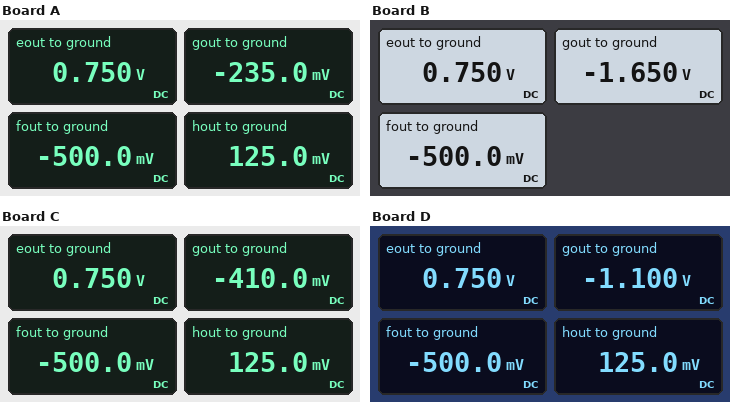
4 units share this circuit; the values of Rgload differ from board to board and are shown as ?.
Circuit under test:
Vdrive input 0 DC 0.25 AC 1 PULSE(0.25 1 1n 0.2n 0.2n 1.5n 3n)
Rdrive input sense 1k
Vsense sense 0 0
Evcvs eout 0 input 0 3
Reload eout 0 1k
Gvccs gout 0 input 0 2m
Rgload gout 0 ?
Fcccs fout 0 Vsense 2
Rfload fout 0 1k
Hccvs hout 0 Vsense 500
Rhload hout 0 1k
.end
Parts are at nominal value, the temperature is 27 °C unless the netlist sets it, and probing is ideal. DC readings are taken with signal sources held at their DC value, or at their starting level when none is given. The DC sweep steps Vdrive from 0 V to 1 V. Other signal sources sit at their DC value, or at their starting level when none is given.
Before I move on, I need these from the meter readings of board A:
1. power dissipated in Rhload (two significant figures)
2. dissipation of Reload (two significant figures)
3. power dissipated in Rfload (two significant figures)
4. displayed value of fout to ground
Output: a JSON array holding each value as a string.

["16 µW", "560 µW", "250 µW", "-500.0 mV"]
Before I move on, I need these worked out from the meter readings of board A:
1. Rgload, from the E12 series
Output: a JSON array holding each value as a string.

["470 Ω"]
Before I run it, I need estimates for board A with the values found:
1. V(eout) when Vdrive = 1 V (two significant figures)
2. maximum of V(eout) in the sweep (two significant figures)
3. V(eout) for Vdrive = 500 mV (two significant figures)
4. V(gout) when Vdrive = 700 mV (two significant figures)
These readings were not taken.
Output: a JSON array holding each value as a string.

["3.0 V", "3.0 V", "1.5 V", "-660 mV"]
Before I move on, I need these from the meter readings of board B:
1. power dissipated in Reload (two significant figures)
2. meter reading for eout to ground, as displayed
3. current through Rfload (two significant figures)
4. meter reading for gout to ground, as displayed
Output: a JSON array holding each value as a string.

["560 µW", "0.750 V", "500 µA", "-1.650 V"]
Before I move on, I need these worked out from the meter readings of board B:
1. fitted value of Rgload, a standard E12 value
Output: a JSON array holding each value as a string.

["3.3 kΩ"]
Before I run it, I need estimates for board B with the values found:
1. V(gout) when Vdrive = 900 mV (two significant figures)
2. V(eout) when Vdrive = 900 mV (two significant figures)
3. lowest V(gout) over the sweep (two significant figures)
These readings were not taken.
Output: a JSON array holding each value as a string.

["-5.9 V", "2.7 V", "-6.6 V"]
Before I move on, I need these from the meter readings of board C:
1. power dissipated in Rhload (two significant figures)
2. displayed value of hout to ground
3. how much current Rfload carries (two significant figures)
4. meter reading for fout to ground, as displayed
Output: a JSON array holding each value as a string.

["16 µW", "125.0 mV", "500 µA", "-500.0 mV"]
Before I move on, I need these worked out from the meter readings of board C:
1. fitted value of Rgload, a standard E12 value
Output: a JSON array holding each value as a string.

["820 Ω"]
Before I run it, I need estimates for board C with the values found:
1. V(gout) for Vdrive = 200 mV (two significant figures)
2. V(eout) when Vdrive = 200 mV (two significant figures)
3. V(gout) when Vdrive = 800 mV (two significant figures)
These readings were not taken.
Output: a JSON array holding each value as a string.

["-330 mV", "600 mV", "-1.3 V"]
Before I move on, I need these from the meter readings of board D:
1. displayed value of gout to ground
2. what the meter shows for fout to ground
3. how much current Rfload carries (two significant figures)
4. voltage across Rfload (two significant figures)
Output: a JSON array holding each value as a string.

["-1.100 V", "-500.0 mV", "500 µA", "500 mV"]
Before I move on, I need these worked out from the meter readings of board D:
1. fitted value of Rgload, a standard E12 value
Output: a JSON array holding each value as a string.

["2.2 kΩ"]
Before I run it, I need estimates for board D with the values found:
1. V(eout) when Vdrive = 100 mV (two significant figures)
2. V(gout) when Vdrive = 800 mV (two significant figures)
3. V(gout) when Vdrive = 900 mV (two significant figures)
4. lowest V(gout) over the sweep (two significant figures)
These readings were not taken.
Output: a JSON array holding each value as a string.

["300 mV", "-3.5 V", "-4.0 V", "-4.4 V"]
